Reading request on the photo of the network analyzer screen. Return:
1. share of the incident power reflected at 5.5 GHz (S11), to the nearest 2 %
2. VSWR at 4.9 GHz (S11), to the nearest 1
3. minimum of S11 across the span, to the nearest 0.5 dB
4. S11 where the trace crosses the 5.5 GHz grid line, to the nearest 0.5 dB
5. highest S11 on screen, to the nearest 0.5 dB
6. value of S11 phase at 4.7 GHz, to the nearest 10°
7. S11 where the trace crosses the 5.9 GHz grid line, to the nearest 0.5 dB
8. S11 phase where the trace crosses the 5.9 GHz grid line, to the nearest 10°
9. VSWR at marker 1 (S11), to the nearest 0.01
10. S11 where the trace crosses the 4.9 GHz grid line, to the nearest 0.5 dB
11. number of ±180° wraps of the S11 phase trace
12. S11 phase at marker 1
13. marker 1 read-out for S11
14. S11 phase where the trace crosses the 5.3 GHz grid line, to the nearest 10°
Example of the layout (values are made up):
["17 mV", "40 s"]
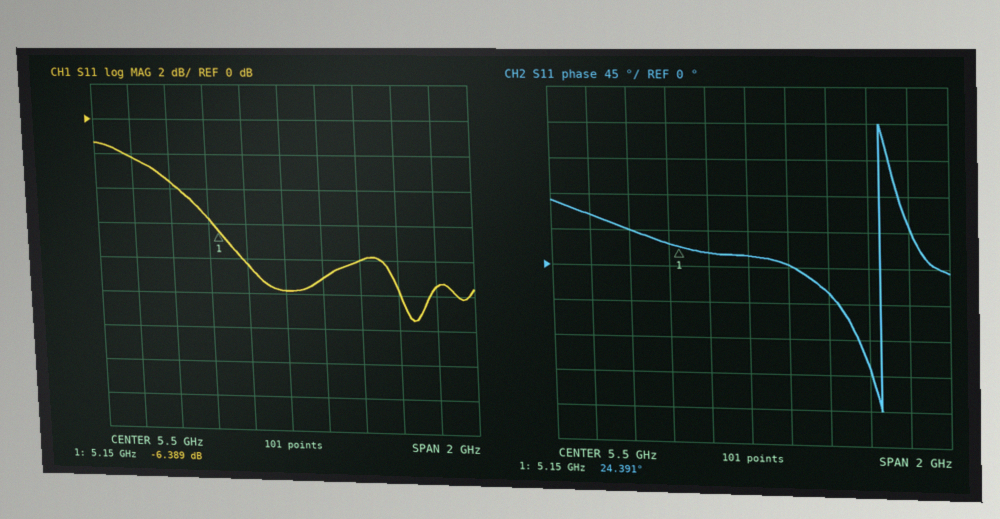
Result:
["10 %", "5", "-11.5 dB", "-10.0 dB", "-1.5 dB", "60°", "-8.0 dB", "-30°", "2.84", "-3.5 dB", "1", "24.391°", "-6.389 dB", "20°"]
